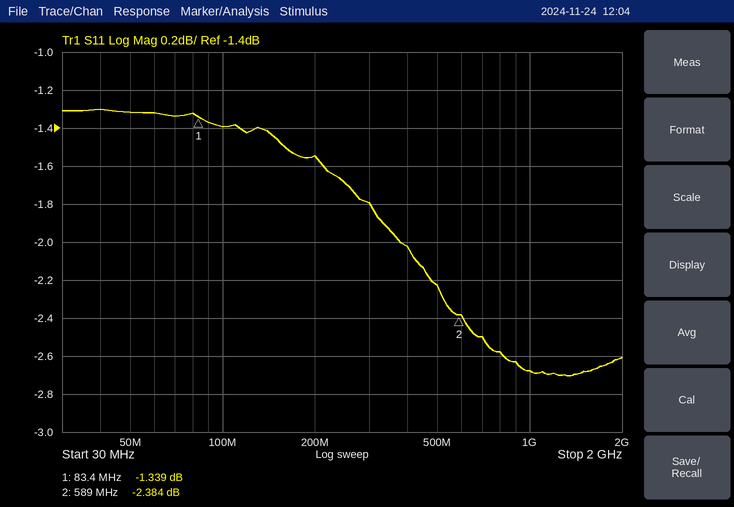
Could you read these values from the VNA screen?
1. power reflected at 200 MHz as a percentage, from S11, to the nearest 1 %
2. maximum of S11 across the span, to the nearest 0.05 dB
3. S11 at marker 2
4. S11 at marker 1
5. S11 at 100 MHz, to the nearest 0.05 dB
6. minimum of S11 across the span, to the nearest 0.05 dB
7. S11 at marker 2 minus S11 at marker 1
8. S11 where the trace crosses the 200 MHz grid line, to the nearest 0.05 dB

70 %
-1.30 dB
-2.384 dB
-1.339 dB
-1.40 dB
-2.70 dB
-1.045 dB
-1.55 dB
